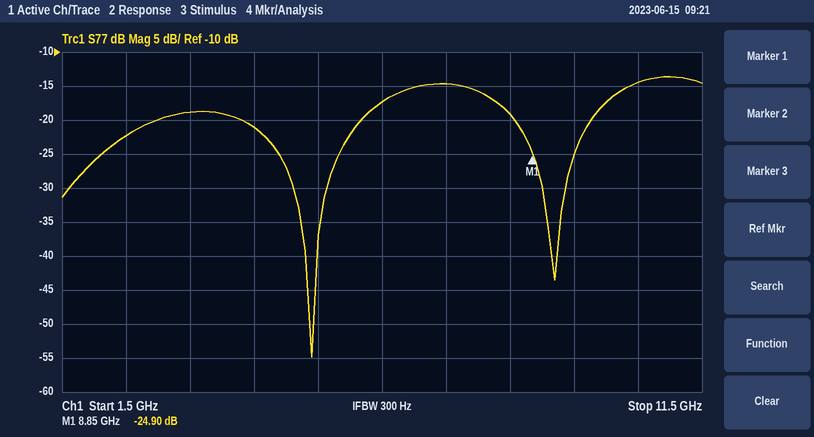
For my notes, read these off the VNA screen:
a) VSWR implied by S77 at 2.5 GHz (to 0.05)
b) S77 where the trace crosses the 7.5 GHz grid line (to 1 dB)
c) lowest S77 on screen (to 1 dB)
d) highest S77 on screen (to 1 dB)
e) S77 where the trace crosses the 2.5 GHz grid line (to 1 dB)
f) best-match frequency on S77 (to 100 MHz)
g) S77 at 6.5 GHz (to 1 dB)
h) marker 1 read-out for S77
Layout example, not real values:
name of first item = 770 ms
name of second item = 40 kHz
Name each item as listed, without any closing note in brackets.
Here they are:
VSWR implied by S77 at 2.5 GHz = 1.15
S77 where the trace crosses the 7.5 GHz grid line = -15 dB
lowest S77 on screen = -55 dB
highest S77 on screen = -14 dB
S77 where the trace crosses the 2.5 GHz grid line = -22 dB
best-match frequency on S77 = 5.4 GHz
S77 at 6.5 GHz = -17 dB
marker 1 read-out for S77 = -24.90 dB
